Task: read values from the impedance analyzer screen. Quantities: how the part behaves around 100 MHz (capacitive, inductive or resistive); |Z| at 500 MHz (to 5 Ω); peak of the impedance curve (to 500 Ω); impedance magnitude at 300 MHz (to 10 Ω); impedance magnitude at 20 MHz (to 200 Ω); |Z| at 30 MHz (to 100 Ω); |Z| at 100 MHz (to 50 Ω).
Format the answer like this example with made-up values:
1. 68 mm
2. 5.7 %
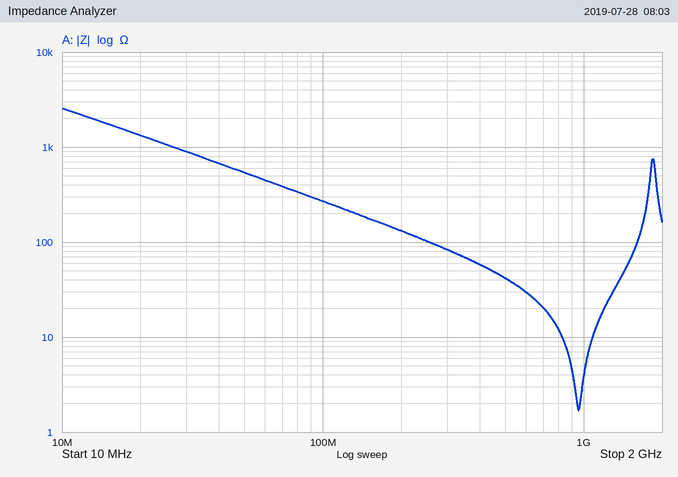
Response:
1. capacitive
2. 40 Ω
3. 2.5 kΩ
4. 80 Ω
5. 1.4 kΩ
6. 900 Ω
7. 250 Ω
